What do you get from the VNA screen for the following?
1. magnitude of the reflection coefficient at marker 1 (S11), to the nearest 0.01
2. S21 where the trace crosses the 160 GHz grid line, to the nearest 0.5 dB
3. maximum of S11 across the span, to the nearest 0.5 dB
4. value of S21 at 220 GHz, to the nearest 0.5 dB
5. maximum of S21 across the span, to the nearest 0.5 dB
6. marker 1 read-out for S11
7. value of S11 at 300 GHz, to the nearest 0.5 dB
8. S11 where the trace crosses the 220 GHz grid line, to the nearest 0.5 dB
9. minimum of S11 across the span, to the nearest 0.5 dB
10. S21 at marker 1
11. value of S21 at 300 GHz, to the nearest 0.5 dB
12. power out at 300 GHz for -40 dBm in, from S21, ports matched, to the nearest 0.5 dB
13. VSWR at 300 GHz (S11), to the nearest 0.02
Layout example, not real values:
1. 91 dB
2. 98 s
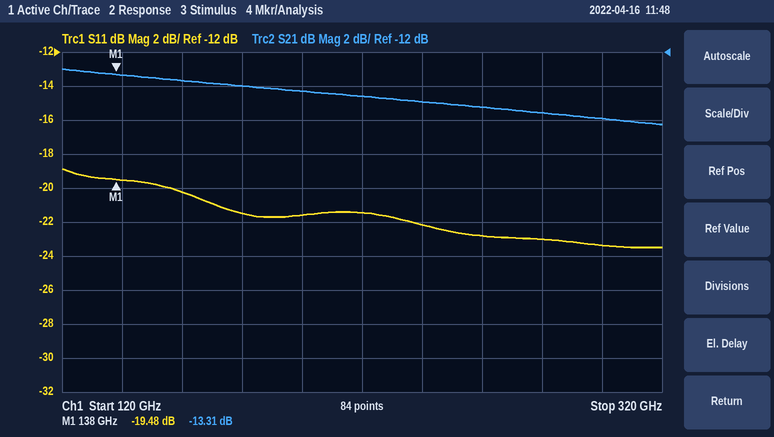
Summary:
1. 0.11
2. -13.5 dB
3. -19.0 dB
4. -14.5 dB
5. -13.0 dB
6. -19.48 dB
7. -23.5 dB
8. -21.5 dB
9. -23.5 dB
10. -13.31 dB
11. -16.0 dB
12. -56.0 dBm
13. 1.14
